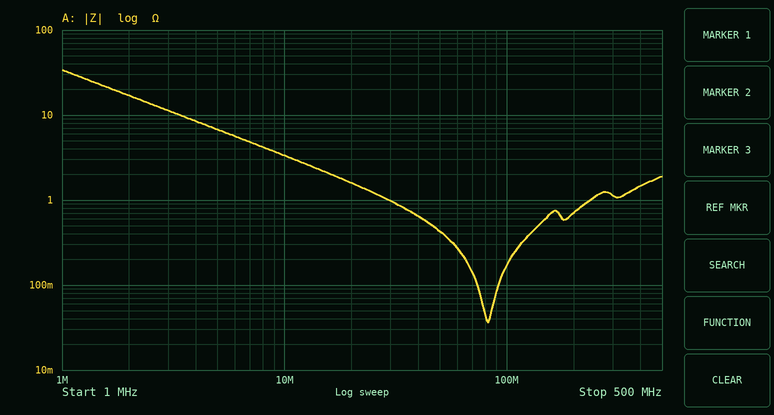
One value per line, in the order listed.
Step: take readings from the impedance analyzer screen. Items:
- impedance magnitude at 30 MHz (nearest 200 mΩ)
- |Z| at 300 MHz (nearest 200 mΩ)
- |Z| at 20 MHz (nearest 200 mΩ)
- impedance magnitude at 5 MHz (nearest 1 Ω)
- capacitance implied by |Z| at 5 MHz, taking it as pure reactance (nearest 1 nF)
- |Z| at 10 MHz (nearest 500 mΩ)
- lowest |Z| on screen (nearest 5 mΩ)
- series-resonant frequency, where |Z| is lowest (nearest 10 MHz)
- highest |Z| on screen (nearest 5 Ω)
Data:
1.0 Ω
1.2 Ω
1.6 Ω
7 Ω
5 nF
3.5 Ω
35 mΩ
80 MHz
35 Ω
